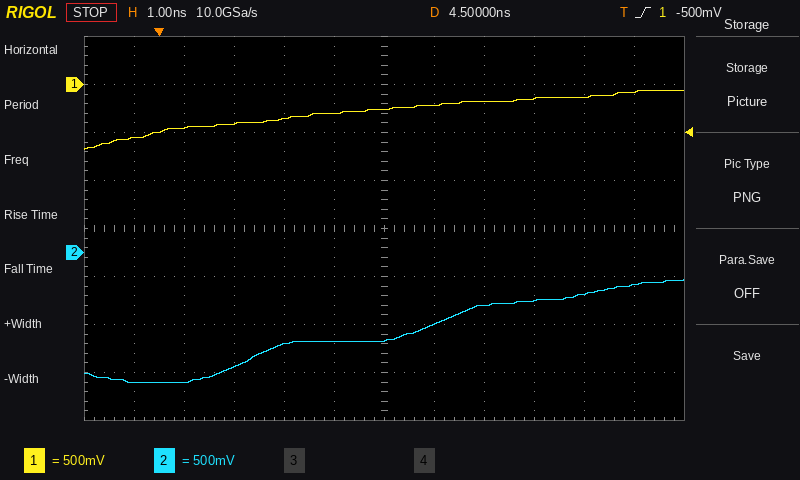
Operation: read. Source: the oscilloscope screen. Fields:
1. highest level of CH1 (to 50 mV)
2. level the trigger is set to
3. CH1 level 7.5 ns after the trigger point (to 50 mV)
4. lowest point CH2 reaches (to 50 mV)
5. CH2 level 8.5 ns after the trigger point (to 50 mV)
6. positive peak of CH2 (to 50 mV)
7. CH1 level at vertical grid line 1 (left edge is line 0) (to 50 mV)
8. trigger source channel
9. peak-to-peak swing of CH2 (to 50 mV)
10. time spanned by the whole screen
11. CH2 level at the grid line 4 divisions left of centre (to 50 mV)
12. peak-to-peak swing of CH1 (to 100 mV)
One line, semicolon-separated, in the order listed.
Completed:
-50 mV; -500 mV; -150 mV; -1.35 V; -450 mV; -300 mV; -550 mV; CH1; 1.05 V; 12 ns; -1.35 V; 600 mV
